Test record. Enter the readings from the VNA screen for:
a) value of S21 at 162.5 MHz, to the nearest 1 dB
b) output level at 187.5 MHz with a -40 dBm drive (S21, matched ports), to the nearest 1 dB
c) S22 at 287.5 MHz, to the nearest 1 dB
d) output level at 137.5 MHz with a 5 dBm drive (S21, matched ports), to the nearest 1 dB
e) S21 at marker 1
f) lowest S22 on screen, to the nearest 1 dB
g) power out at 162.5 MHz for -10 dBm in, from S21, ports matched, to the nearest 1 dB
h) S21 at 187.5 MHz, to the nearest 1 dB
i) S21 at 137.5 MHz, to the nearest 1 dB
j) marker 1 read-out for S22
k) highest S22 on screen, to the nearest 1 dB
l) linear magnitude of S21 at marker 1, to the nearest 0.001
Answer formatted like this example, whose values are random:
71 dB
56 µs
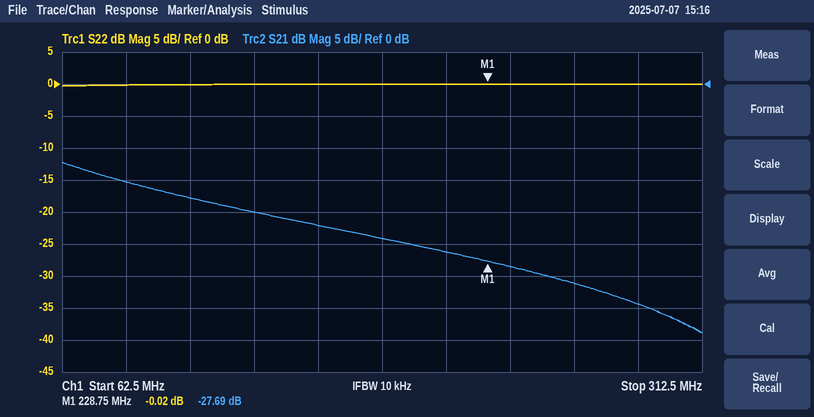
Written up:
-22 dB
-64 dBm
0 dB
-15 dBm
-27.69 dB
0 dB
-32 dBm
-24 dB
-20 dB
-0.02 dB
0 dB
0.041
